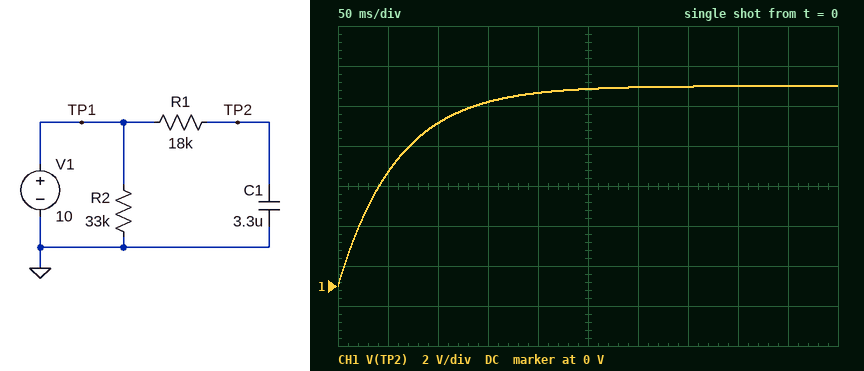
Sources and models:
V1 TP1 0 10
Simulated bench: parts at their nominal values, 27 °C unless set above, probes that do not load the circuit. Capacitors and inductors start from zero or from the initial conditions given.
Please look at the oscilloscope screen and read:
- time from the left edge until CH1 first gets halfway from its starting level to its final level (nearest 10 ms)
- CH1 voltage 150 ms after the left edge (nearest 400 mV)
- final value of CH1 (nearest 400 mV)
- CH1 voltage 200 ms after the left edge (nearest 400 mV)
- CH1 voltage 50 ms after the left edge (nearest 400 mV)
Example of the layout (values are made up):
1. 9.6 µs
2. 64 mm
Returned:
1. 40 ms
2. 9.2 V
3. 10.0 V
4. 9.6 V
5. 5.6 V
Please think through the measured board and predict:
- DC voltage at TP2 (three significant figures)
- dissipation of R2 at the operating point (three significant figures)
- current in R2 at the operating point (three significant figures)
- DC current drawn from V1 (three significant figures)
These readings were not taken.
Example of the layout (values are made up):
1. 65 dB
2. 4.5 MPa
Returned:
1. 10.0 V
2. 3.03 mW
3. 303 µA
4. 303 µA
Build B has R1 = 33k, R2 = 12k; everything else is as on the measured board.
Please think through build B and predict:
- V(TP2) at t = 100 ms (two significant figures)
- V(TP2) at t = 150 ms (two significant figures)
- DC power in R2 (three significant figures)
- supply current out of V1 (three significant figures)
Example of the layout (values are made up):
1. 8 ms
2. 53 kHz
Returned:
1. 6.0 V
2. 7.5 V
3. 8.33 mW
4. 833 µA
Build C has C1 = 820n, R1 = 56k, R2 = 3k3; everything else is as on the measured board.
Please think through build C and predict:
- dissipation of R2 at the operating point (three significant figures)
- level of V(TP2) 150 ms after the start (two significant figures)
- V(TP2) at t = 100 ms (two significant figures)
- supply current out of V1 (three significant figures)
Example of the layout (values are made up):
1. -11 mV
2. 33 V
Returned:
1. 30.3 mW
2. 9.6 V
3. 8.9 V
4. 3.03 mA
